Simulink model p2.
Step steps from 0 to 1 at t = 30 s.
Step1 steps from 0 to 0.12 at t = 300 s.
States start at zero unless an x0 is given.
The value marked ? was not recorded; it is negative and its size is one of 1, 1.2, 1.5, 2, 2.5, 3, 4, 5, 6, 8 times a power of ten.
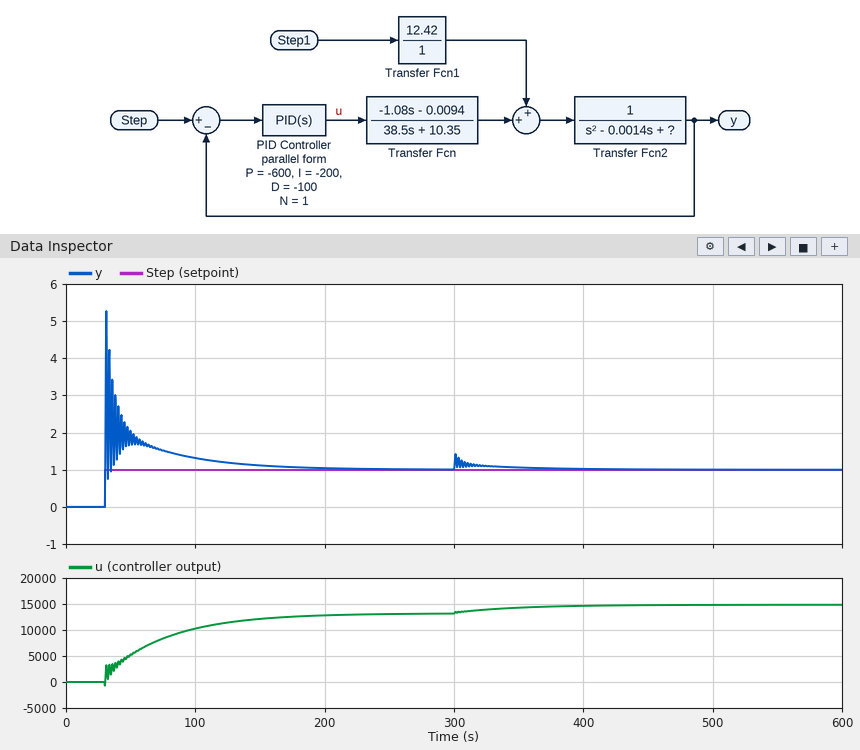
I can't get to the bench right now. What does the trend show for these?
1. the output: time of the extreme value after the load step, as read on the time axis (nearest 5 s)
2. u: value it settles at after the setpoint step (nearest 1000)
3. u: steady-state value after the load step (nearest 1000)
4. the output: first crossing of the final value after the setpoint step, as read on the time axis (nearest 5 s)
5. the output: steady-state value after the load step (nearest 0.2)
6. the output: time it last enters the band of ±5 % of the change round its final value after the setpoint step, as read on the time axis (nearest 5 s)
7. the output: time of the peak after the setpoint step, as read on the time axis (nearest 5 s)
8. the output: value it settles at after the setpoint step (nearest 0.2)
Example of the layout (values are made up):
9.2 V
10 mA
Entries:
300 s
13000
15000
30 s
1.0
190 s
30 s
1.0
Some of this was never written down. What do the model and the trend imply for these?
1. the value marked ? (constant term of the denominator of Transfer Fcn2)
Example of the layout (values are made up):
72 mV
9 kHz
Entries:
-12
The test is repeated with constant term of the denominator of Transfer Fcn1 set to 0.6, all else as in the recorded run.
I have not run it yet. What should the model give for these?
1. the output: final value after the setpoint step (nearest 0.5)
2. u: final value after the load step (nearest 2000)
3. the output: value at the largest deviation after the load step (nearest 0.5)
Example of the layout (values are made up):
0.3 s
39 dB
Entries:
1.0
16000
1.5
